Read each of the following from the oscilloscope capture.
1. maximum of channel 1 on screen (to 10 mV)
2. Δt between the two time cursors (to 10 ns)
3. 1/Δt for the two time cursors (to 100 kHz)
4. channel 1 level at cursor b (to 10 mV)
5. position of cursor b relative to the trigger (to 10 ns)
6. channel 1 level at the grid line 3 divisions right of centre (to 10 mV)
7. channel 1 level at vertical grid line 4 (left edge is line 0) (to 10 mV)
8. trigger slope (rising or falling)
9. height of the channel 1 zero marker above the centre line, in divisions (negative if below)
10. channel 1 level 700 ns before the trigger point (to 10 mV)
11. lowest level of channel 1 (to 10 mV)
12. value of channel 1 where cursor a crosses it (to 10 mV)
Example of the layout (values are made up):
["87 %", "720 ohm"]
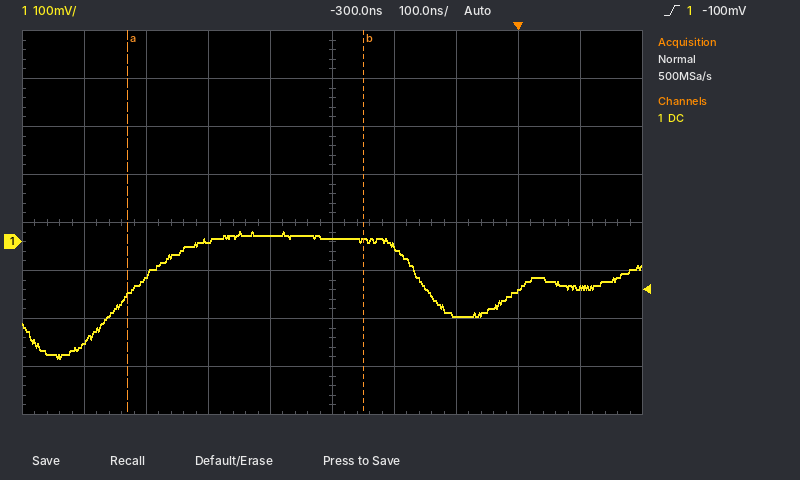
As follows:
["20 mV", "380 ns", "2.6 MHz", "0 mV", "-250 ns", "-100 mV", "10 mV", "rising", "-0.4 div", "-210 mV", "-240 mV", "-110 mV"]
